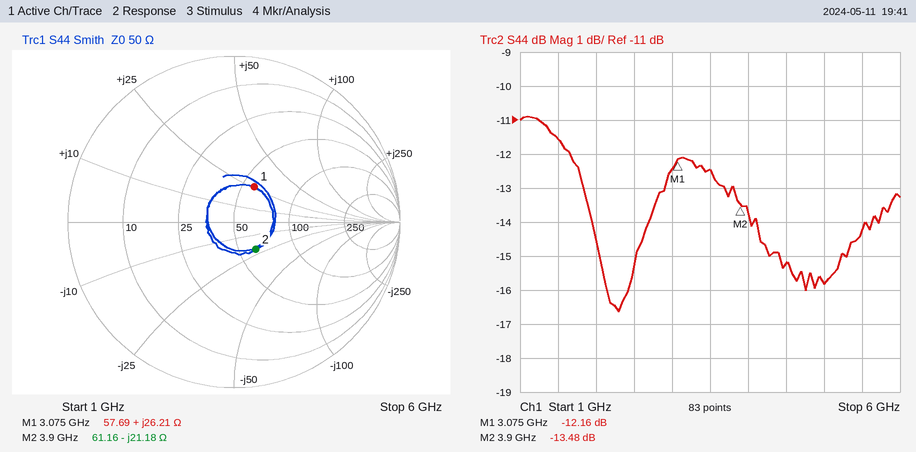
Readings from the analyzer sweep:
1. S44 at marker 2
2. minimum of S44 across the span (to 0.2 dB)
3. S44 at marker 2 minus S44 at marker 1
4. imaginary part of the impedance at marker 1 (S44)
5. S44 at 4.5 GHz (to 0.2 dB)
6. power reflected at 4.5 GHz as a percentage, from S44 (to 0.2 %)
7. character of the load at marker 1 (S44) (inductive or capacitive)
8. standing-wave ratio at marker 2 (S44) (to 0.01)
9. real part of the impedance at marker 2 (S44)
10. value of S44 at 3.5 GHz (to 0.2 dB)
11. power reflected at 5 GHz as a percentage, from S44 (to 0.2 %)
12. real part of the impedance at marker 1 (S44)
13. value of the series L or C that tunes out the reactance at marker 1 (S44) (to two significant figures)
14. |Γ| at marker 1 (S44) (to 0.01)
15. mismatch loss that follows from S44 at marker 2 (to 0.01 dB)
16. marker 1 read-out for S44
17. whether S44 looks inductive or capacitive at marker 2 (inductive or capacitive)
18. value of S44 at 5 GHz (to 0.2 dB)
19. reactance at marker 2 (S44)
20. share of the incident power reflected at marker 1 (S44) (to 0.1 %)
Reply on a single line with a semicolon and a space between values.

-13.48 dB; -16.6 dB; -1.32 dB; +26.21 Ω; -15.2 dB; 3.0 %; inductive; 1.54; 61.16 Ω; -12.4 dB; 2.6 %; 57.69 Ω; 2.0 pF; 0.25; 0.20 dB; -12.16 dB; capacitive; -15.8 dB; -21.18 Ω; 6.1 %
